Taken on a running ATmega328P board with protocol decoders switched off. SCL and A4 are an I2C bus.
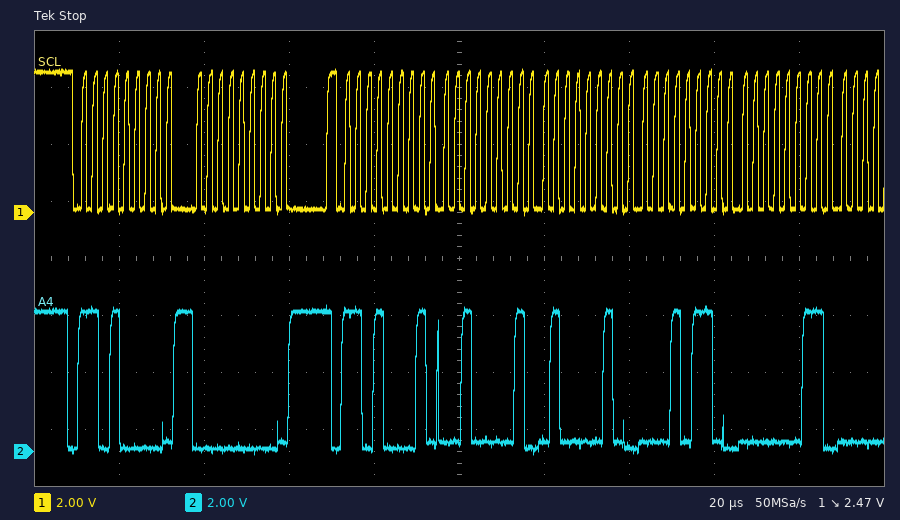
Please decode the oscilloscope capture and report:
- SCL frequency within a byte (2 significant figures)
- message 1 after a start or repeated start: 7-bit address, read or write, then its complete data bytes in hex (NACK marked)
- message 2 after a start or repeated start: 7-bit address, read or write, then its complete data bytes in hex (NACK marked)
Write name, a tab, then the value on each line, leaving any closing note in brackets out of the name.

SCL frequency within a byte	400 kHz
message 1 after a start or repeated start: 7-bit address, read or write, then its complete data bytes in hex	0x68 write: 00
message 2 after a start or repeated start: 7-bit address, read or write, then its complete data bytes in hex	0x68 read: 21 42 16 03
